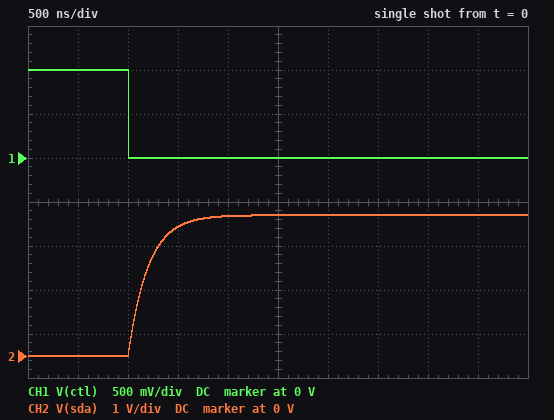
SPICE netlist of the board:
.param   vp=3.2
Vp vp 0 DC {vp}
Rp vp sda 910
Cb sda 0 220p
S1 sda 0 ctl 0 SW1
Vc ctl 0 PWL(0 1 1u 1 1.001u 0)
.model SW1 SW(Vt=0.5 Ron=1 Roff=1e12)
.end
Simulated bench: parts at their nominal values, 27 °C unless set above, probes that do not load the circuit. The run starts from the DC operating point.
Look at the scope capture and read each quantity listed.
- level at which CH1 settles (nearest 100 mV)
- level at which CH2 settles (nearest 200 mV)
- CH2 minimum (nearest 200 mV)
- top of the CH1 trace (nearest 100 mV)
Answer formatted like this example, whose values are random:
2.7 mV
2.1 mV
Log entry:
0 V
3.2 V
0 V
1.0 V
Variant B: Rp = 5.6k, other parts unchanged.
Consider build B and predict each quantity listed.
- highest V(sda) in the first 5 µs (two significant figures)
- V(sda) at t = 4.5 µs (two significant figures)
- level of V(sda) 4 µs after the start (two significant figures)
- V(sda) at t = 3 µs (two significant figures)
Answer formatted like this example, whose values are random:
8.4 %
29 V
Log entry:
3.1 V
3.0 V
2.9 V
2.6 V
